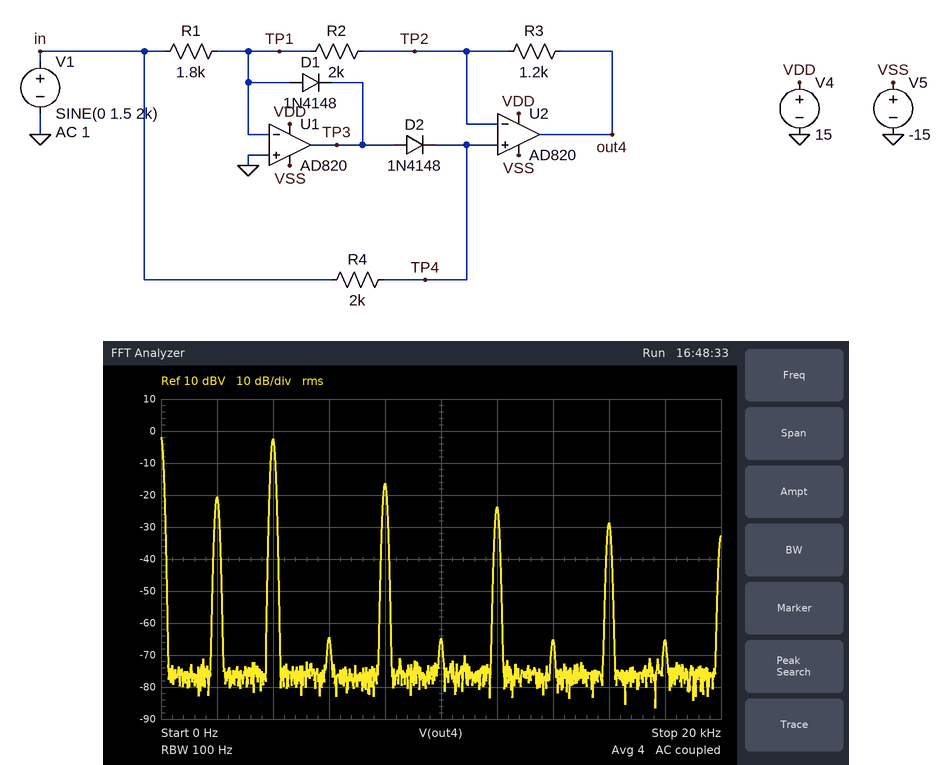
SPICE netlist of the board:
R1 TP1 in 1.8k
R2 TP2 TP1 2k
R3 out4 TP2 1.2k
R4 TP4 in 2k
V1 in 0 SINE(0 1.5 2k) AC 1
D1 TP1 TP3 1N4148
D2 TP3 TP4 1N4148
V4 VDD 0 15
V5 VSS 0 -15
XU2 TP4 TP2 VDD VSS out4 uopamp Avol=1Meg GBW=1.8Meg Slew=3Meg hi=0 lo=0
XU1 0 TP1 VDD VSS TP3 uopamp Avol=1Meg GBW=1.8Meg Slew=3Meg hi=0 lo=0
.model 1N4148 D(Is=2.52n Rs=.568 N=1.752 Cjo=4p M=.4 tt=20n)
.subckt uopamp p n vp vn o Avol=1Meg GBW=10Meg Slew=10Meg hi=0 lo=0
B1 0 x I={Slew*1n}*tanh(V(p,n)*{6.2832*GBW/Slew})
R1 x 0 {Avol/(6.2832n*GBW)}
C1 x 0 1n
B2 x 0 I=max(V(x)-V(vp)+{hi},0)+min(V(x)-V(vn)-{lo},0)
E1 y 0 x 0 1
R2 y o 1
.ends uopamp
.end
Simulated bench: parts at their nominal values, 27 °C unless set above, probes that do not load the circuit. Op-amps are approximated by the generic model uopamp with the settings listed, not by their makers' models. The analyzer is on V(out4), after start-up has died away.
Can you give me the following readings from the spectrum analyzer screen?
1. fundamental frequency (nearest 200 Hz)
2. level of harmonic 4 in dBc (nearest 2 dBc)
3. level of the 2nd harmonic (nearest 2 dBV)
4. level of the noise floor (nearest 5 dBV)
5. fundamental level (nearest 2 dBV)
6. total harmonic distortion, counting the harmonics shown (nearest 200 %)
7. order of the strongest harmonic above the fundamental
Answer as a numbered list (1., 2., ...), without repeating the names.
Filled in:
1. 2.0 kHz
2. 4 dBc
3. -2 dBV
4. -75 dBV
5. -20 dBV
6. 800 %
7. 2
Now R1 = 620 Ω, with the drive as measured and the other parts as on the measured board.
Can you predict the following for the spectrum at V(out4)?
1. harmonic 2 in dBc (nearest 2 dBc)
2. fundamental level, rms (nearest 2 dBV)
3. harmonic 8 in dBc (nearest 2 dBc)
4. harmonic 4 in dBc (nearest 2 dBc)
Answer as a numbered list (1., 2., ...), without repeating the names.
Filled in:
1. -2 dBc
2. 6 dBV
3. -28 dBc
4. -16 dBc
